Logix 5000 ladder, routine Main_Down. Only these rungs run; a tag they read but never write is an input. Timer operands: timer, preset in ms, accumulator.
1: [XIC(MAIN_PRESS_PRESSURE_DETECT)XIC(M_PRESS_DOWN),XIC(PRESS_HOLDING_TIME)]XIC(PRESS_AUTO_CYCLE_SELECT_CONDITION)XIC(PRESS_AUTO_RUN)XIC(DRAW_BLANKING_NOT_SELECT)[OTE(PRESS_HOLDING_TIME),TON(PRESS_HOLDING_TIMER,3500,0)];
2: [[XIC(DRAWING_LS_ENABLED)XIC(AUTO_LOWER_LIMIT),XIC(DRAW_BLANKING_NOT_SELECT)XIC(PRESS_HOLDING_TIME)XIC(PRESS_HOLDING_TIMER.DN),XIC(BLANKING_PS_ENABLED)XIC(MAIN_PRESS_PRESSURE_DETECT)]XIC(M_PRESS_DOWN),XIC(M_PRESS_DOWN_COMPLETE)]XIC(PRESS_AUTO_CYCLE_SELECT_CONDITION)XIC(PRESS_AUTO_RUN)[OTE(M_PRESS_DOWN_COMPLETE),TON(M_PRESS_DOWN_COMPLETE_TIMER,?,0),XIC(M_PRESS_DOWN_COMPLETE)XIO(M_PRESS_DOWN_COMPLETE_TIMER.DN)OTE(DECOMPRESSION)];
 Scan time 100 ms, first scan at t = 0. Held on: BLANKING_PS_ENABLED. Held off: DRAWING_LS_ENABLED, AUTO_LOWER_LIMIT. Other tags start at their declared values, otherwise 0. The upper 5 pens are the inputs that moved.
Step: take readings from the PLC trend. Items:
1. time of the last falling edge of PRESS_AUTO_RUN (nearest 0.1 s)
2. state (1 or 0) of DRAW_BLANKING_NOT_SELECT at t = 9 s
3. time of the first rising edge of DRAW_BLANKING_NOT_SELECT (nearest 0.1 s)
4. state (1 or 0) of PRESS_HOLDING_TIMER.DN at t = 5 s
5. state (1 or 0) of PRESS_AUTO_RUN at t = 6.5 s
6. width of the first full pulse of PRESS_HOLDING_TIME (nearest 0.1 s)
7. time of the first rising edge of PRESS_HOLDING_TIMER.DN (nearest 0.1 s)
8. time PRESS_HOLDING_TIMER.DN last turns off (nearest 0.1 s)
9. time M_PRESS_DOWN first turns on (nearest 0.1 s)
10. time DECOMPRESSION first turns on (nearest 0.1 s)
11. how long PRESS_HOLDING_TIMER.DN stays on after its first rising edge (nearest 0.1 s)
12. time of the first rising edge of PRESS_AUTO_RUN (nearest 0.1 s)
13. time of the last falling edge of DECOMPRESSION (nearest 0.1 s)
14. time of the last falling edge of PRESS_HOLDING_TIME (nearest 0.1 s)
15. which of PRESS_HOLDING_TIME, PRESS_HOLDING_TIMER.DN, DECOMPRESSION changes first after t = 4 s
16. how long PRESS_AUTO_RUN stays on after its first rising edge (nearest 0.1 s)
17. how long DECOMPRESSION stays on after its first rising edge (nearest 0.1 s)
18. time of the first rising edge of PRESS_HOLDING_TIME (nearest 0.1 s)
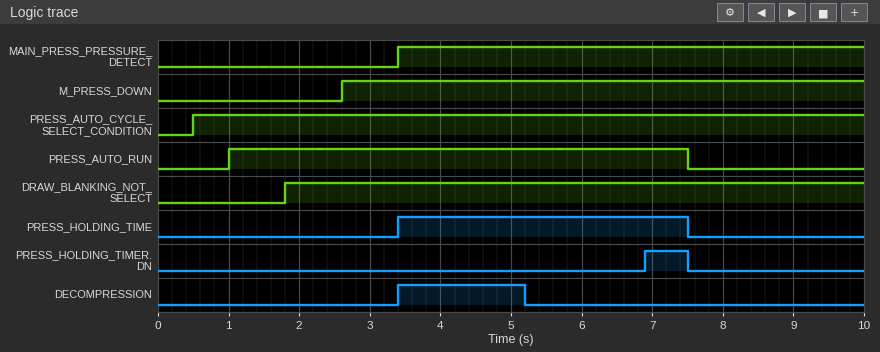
7.5 s
1
1.8 s
0
1
4.1 s
6.9 s
7.5 s
2.6 s
3.4 s
0.6 s
1.0 s
5.2 s
7.5 s
DECOMPRESSION
6.5 s
1.8 s
3.4 s
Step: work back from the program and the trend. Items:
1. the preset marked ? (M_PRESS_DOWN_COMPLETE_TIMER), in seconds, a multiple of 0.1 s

1.8 s
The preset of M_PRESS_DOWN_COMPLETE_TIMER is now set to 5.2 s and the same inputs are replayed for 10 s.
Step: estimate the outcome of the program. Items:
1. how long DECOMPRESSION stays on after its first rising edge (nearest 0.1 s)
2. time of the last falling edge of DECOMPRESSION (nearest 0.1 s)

4.1 s
7.5 s
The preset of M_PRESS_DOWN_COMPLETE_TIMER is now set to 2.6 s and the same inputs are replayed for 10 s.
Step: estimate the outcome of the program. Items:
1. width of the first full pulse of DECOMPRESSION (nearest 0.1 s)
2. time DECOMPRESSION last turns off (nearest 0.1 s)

2.6 s
6.0 s
